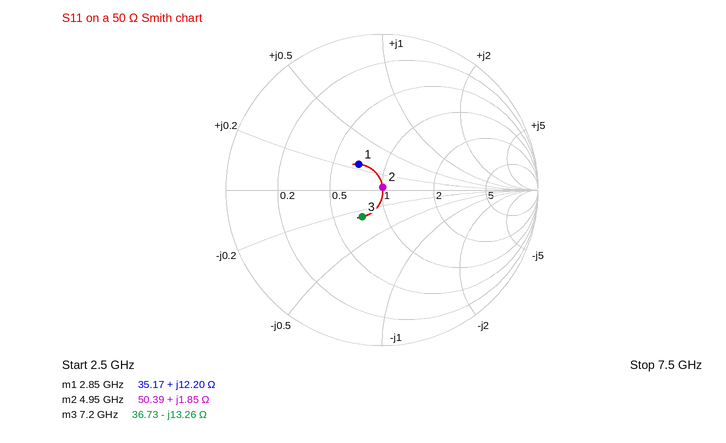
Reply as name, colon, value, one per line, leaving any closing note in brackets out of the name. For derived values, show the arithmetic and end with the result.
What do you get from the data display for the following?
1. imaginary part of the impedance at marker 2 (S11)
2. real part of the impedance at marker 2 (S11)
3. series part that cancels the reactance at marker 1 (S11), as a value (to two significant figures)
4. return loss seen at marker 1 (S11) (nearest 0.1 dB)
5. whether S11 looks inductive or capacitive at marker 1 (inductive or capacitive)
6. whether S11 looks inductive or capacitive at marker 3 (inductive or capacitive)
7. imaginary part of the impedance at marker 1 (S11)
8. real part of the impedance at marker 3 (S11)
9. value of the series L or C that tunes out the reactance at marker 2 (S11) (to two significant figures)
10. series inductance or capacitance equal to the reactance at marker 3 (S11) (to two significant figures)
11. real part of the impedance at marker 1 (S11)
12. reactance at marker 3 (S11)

imaginary part of the impedance at marker 2: +1.85 Ω
real part of the impedance at marker 2: 50.39 Ω
series part that cancels the reactance at marker 1 (S11), as a value: C = 1/(2π × 2.85 GHz × 12.2 Ω) ≈ 4.6 pF
return loss seen at marker 1 (S11): 13.0 dB
whether S11 looks inductive or capacitive at marker 1: inductive
whether S11 looks inductive or capacitive at marker 3: capacitive
imaginary part of the impedance at marker 1: +12.20 Ω
real part of the impedance at marker 3: 36.73 Ω
value of the series L or C that tunes out the reactance at marker 2 (S11): C = 1/(2π × 4.95 GHz × 1.85 Ω) ≈ 17 pF
series inductance or capacitance equal to the reactance at marker 3 (S11): C = 1/(2π × 7.2 GHz × 13.26 Ω) ≈ 1.7 pF
real part of the impedance at marker 1: 35.17 Ω
reactance at marker 3: -13.26 Ω
